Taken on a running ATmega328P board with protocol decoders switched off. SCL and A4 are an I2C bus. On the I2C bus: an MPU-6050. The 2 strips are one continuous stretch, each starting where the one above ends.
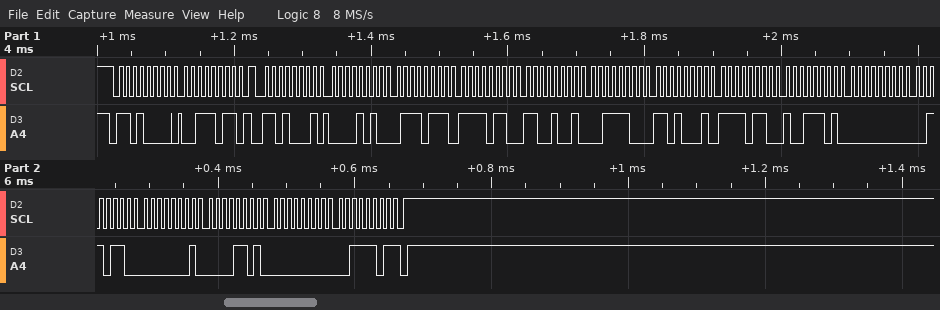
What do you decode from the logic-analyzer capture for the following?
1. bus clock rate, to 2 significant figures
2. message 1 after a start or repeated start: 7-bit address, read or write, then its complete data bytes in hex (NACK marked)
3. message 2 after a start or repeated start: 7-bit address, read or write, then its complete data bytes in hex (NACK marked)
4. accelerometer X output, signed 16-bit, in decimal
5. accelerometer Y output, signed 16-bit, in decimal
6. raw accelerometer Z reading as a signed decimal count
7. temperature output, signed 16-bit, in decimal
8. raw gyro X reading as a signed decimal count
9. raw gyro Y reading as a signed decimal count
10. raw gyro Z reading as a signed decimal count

100 kHz
0x68 write: 3B
0x68 read: 0A 77 F6 C9 3C D1 F6 9D 00 36 01 0D 00 3D NACK
2679
-2359
15569
-2403
54
269
61
